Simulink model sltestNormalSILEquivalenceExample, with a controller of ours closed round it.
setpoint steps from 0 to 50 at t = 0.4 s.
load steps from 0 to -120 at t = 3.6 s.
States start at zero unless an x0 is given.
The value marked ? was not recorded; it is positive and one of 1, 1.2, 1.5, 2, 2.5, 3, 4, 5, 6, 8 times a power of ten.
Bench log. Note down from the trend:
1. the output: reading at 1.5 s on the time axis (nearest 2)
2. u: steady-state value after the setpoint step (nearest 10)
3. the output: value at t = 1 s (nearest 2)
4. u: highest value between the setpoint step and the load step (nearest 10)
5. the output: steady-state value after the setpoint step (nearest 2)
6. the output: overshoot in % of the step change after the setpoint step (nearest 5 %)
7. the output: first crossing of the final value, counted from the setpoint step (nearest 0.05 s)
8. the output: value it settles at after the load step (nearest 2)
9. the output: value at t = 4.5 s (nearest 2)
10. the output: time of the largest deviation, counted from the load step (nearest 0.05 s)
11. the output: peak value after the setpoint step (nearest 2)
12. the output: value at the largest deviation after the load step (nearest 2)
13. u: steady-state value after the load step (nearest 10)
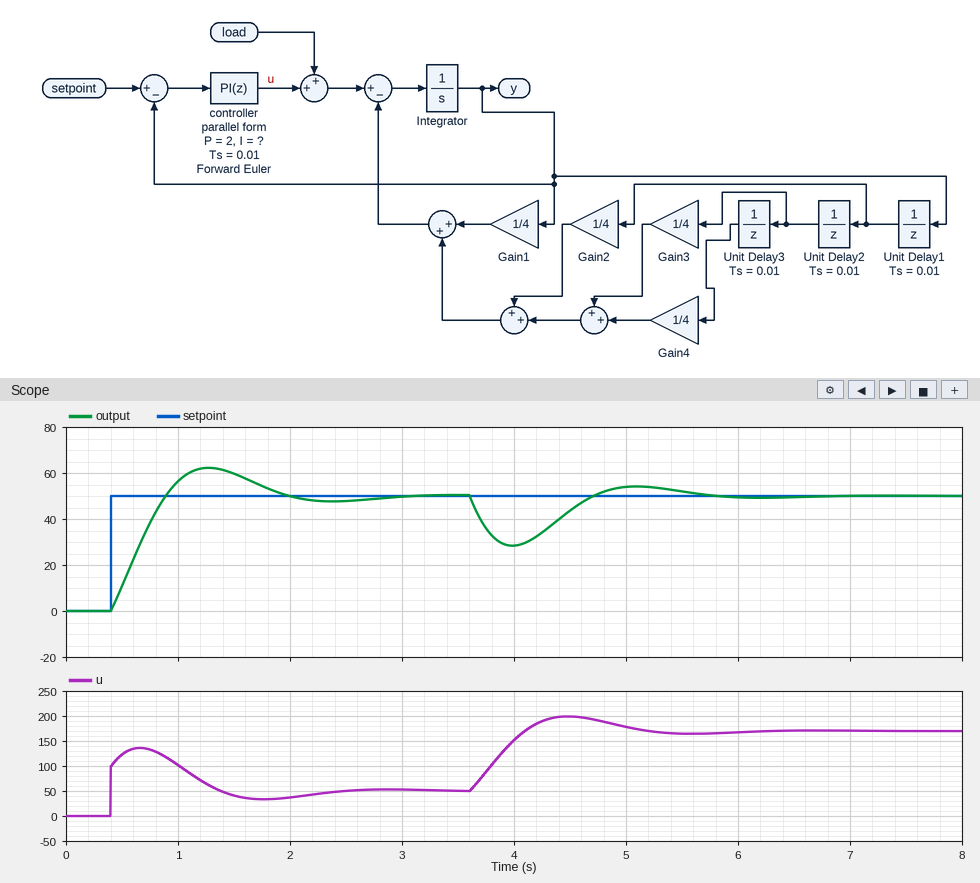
60
50
56
140
50
25 %
0.50 s
50
44
0.40 s
62
28
170
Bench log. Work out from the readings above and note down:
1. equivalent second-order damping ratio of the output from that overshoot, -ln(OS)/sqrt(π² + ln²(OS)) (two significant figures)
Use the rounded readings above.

0.40
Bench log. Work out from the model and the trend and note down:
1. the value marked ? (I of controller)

10
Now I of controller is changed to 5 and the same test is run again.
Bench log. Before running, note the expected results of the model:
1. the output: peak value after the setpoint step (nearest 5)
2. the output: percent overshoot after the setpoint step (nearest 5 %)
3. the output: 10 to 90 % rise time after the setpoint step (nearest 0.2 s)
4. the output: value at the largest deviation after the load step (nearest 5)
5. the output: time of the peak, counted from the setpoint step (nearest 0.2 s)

55
10 %
0.6 s
25
1.2 s
